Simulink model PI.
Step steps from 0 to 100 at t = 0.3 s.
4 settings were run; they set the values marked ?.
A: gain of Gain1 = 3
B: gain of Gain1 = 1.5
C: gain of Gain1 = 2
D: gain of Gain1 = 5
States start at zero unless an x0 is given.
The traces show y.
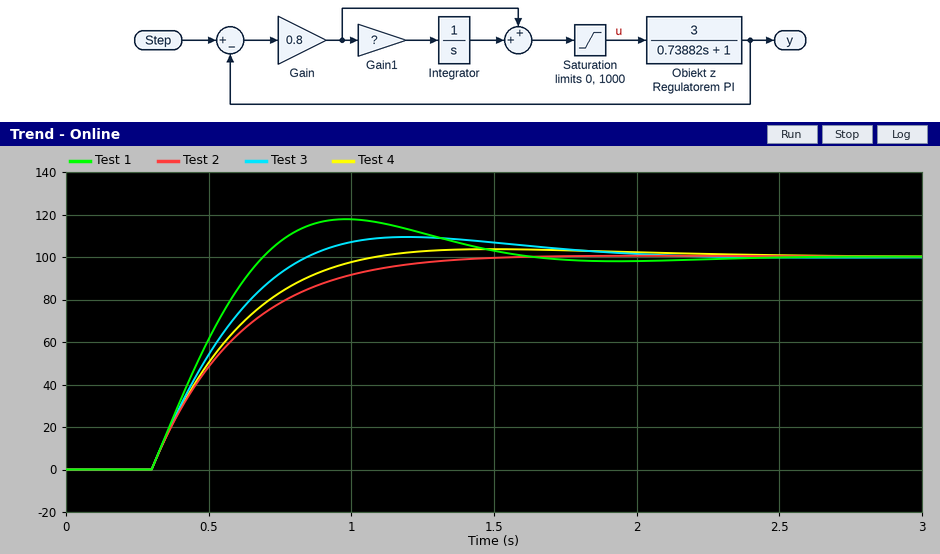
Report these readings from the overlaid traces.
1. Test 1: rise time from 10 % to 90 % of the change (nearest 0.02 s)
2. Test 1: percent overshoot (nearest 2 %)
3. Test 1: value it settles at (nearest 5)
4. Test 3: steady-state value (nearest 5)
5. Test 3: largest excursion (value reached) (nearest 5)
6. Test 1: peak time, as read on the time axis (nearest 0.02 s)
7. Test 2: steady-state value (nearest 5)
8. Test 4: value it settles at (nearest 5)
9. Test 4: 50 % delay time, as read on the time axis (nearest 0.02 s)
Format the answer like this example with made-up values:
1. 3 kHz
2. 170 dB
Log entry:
1. 0.30 s
2. 18 %
3. 100
4. 100
5. 110
6. 0.98 s
7. 100
8. 100
9. 0.50 s
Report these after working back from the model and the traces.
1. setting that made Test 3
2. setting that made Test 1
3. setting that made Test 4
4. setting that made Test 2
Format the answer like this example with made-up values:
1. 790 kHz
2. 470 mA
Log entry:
1. A
2. D
3. C
4. B
